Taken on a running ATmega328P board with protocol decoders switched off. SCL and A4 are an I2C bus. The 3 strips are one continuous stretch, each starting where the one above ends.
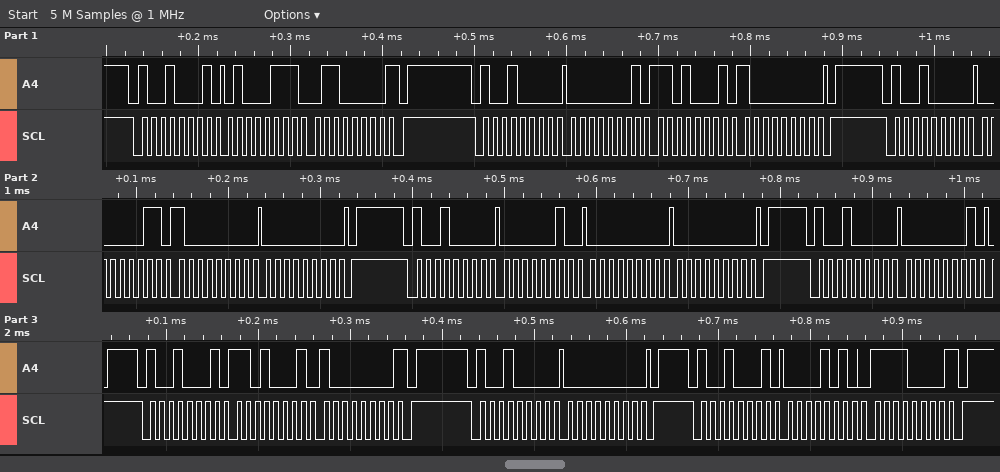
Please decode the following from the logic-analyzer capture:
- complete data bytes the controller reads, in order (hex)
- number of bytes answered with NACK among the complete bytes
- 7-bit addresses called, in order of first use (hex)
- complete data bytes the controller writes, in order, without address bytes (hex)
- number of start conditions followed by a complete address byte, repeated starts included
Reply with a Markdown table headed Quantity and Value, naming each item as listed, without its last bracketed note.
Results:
| Quantity | Value |
|---|---|
| complete data bytes the controller reads, in order | 47 60 D1 80 0A F0 |
| number of bytes answered with NACK among the complete bytes | 3 |
| 7-bit addresses called, in order of first use | 0x48 |
| complete data bytes the controller writes, in order, without address bytes | 01 D1 80 03 80 00 02 00 00 01 00 |
| number of start conditions followed by a complete address byte, repeated starts included | 8 |
